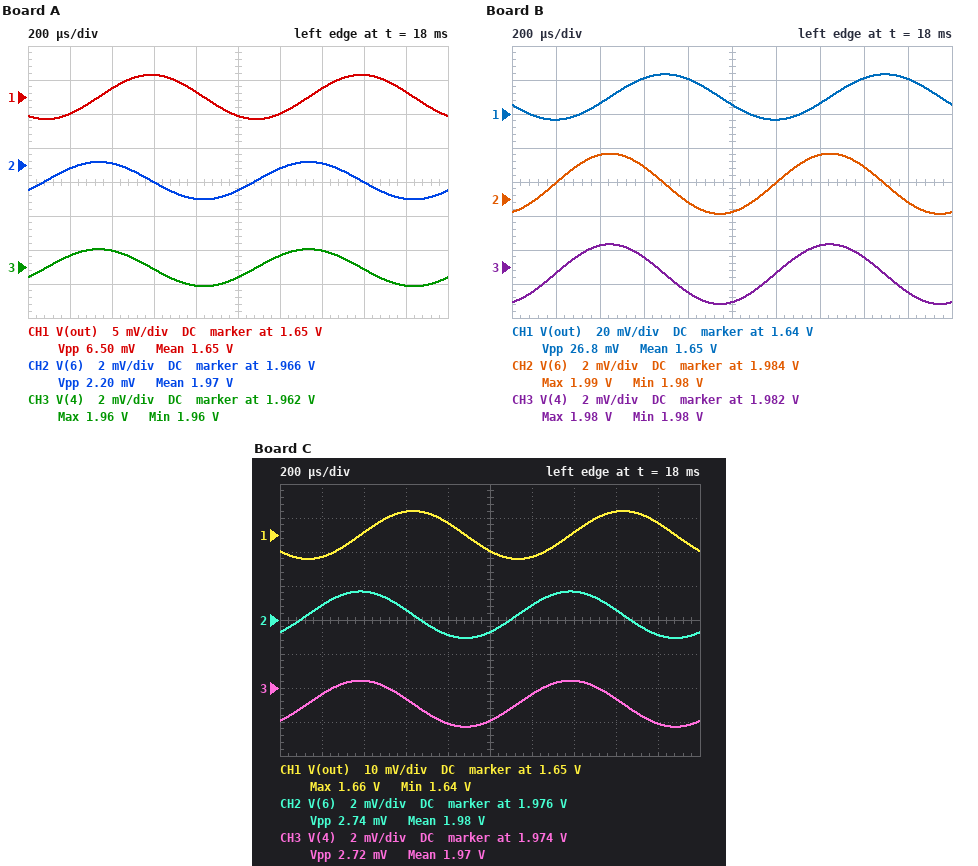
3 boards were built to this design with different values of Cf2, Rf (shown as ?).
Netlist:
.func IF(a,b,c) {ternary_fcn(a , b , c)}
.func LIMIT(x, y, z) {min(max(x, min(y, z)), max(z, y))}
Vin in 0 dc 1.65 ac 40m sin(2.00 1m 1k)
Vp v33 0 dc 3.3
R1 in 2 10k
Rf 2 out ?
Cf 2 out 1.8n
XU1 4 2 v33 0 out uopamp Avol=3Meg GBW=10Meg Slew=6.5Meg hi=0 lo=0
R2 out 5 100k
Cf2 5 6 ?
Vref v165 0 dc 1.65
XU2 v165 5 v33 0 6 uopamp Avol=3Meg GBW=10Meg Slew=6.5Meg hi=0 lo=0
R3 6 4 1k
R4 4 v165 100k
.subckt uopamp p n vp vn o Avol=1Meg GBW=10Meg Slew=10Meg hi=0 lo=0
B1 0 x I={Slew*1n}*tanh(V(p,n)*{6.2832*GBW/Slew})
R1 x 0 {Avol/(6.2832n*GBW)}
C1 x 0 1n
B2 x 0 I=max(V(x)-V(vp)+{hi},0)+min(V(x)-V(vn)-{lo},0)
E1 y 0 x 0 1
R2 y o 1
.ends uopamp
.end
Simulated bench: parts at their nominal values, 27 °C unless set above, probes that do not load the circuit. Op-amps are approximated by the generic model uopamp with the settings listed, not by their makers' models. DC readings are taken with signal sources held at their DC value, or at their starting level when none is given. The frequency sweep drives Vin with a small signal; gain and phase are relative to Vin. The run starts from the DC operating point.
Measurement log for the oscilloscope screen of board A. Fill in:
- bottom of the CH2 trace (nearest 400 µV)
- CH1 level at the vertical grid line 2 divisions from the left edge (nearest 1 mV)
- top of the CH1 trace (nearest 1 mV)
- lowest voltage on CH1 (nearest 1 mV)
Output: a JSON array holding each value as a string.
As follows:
["1.9640 V", "1.651 V", "1.653 V", "1.647 V"]
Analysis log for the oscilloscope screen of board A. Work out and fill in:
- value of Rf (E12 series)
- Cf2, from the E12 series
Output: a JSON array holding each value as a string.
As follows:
["82 kΩ", "4.7 nF"]
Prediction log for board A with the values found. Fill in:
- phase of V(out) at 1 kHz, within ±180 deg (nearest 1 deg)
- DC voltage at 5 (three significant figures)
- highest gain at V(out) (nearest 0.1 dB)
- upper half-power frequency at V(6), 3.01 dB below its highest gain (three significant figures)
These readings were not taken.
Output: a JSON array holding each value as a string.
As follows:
["-121 deg", "1.65 V", "15.9 dB", "2.17 kHz"]
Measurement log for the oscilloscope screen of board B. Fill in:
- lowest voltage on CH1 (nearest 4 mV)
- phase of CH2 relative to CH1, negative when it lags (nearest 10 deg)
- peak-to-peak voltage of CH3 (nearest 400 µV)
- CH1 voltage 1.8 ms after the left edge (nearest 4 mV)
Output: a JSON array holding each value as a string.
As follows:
["1.636 V", "90 deg", "3.6 mV", "1.660 V"]
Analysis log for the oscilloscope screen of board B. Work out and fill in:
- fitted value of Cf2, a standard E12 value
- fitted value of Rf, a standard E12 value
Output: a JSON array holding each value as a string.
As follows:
["12 nF", "180 kΩ"]
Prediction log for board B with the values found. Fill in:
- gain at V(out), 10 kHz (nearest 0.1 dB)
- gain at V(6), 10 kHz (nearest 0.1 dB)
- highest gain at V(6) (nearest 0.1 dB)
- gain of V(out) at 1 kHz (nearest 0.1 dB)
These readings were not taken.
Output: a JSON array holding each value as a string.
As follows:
["-1.0 dB", "-38.5 dB", "5.0 dB", "22.5 dB"]
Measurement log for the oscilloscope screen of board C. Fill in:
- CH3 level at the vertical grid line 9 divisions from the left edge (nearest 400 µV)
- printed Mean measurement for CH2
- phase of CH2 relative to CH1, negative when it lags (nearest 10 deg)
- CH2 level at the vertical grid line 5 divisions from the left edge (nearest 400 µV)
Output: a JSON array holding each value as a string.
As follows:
["1.9720 V", "1.98 V", "90 deg", "1.9752 V"]
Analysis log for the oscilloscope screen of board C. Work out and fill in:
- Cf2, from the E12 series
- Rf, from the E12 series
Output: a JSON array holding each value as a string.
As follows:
["8.2 nF", "120 kΩ"]
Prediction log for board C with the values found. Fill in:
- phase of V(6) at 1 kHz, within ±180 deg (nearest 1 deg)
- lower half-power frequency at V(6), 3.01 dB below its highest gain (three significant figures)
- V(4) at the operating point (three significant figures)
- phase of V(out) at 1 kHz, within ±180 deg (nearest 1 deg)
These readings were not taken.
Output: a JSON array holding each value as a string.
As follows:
["-48 deg", "476 Hz", "1.65 V", "-138 deg"]
